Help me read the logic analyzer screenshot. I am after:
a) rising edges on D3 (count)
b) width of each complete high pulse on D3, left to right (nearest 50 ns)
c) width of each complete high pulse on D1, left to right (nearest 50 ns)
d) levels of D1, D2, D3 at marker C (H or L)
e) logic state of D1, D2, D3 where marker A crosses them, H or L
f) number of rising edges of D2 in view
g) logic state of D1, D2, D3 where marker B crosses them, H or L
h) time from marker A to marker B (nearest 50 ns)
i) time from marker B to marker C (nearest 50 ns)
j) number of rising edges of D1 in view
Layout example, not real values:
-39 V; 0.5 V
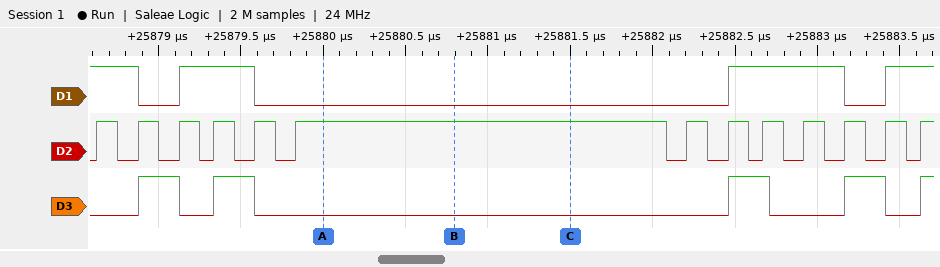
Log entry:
5; 250 ns, 250 ns, 250 ns, 250 ns; 450 ns, 700 ns; D1=L, D2=H, D3=L; D1=L, D2=H, D3=L; 13; D1=L, D2=H, D3=L; 800 ns; 700 ns; 3
